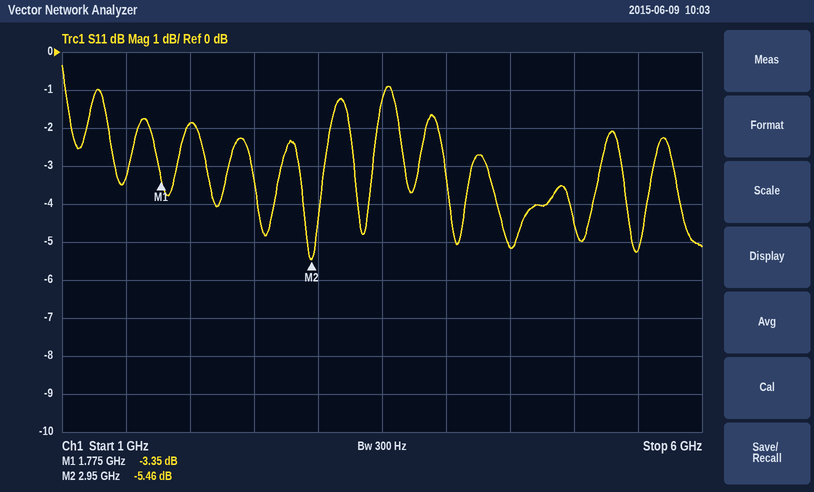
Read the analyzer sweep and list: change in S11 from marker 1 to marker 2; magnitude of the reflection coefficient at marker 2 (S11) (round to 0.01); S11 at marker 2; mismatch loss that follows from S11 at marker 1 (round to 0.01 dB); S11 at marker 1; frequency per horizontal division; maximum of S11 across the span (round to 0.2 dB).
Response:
-2.11 dB
0.53
-5.46 dB
2.70 dB
-3.35 dB
500 MHz
-0.4 dB
